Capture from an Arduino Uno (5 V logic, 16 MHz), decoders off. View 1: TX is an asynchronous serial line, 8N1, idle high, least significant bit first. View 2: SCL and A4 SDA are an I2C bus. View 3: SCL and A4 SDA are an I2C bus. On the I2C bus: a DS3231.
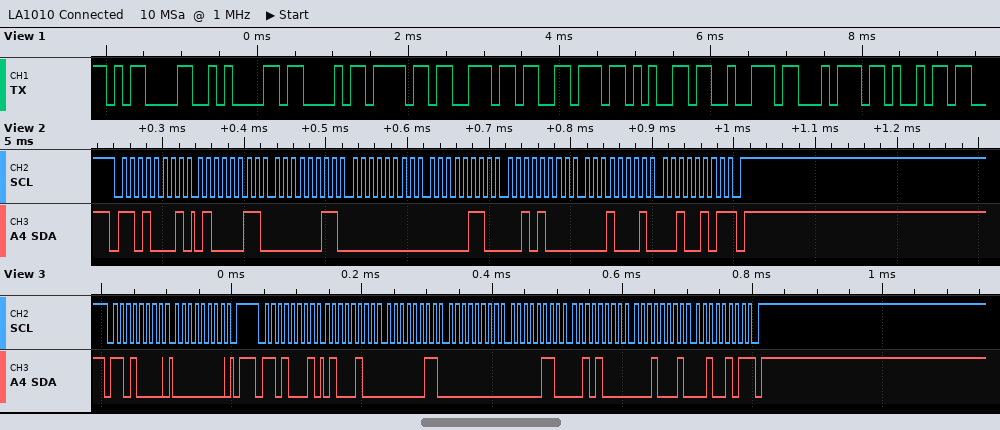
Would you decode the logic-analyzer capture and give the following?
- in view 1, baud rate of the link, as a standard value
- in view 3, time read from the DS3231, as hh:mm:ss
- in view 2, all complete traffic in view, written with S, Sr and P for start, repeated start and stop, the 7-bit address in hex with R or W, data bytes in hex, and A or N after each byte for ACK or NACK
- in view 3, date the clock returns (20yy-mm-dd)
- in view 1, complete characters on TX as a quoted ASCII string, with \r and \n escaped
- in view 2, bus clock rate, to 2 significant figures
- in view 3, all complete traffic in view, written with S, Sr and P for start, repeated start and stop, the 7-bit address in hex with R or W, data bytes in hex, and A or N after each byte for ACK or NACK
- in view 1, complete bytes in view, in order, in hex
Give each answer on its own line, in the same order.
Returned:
9600 baud
00:03:44
S 68R A 43 A 03 A 00 A 06 A 28 A 11 A 25 N P
2025-11-28
"\r\nConverti"
100 kHz
S 68W A 00 A P S 68R A 44 A 03 A 00 A 06 A 28 A 11 A 25 N P
0D 0A 43 6F 6E 76 65 72 74 69
